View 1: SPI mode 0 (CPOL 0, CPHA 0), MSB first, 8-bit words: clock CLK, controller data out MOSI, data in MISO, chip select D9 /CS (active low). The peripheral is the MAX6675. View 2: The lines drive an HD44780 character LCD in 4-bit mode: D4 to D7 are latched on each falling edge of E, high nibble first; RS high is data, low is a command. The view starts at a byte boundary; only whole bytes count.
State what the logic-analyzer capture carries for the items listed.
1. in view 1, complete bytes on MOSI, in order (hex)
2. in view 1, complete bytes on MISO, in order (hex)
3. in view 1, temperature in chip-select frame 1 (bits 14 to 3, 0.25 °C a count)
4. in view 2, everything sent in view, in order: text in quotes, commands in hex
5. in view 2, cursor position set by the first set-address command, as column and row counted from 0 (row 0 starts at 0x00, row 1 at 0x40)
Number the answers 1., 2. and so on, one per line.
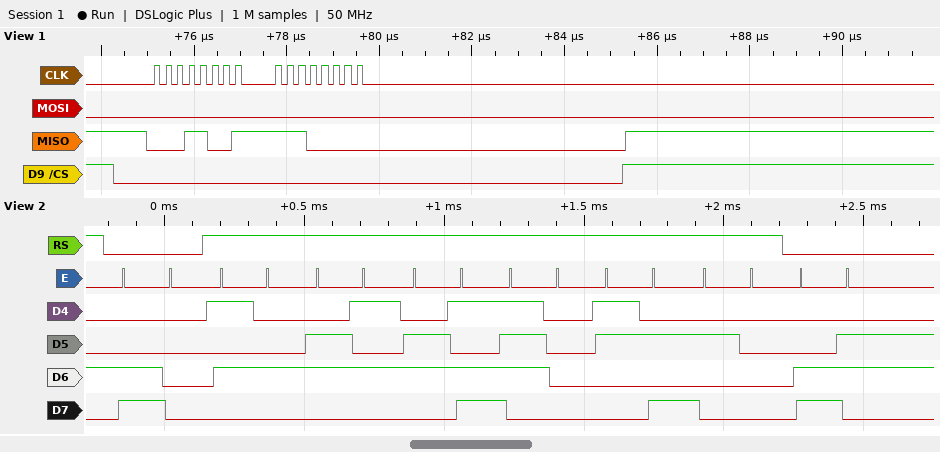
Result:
1. 00 00
2. 19 E0
3. 207.00 °C
4. 0xC0 "Temp: " 0xC6
5. column 0, row 1
